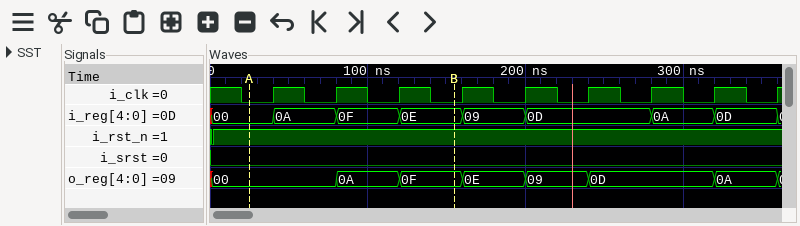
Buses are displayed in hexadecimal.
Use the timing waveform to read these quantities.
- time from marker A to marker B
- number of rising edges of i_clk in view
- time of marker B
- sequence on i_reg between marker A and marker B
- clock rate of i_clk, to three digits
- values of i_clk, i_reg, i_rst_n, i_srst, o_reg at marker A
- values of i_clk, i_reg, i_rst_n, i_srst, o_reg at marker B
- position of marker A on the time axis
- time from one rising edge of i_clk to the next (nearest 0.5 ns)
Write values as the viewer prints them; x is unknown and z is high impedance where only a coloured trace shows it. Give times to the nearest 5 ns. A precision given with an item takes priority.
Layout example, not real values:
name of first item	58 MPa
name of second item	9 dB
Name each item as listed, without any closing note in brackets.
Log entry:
time from marker A to marker B	130 ns
number of rising edges of i_clk in view	9
time of marker B	155 ns
sequence on i_reg between marker A and marker B	00, 0A, 0F, 0E
clock rate of i_clk, to three digits	25.0 MHz
values of i_clk, i_reg, i_rst_n, i_srst, o_reg at marker A	i_clk=0, i_reg=00, i_rst_n=1, i_srst=0, o_reg=00
values of i_clk, i_reg, i_rst_n, i_srst, o_reg at marker B	i_clk=0, i_reg=0E, i_rst_n=1, i_srst=0, o_reg=0F
position of marker A on the time axis	25 ns
time from one rising edge of i_clk to the next	40 ns
